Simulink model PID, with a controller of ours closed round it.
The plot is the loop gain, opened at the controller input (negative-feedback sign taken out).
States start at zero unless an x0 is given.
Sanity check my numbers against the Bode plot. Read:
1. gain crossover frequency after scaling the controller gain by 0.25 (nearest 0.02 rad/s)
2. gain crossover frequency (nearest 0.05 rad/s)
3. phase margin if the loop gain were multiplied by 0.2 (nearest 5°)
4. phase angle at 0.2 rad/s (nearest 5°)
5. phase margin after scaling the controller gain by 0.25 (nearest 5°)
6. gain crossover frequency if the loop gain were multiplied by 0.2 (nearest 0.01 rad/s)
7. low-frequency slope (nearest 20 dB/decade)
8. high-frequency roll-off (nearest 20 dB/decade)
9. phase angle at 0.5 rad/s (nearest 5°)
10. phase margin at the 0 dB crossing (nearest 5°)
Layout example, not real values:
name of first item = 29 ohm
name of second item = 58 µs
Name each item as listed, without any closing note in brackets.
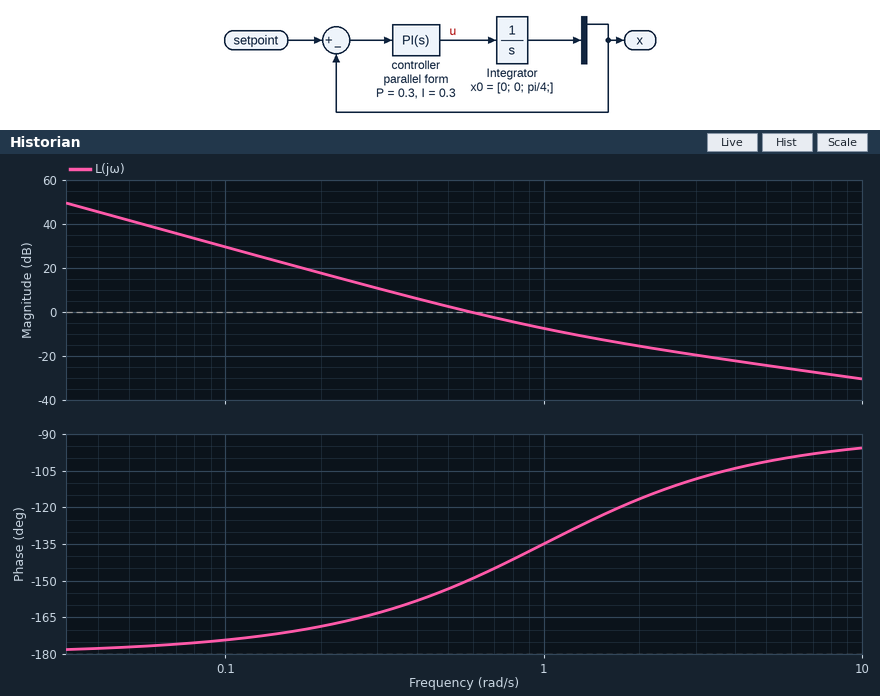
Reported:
gain crossover frequency after scaling the controller gain by 0.25 = 0.28 rad/s
gain crossover frequency = 0.60 rad/s
phase margin if the loop gain were multiplied by 0.2 = 15°
phase angle at 0.2 rad/s = -170°
phase margin after scaling the controller gain by 0.25 = 15°
gain crossover frequency if the loop gain were multiplied by 0.2 = 0.25 rad/s
low-frequency slope = -40 dB/decade
high-frequency roll-off = -20 dB/decade
phase angle at 0.5 rad/s = -155°
phase margin at the 0 dB crossing = 30°
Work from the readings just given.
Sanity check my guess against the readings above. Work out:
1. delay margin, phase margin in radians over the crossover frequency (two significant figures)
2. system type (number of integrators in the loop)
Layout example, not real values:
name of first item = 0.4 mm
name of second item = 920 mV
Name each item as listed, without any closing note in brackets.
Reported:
delay margin, phase margin in radians over the crossover frequency = 0.87 s
system type = 2
